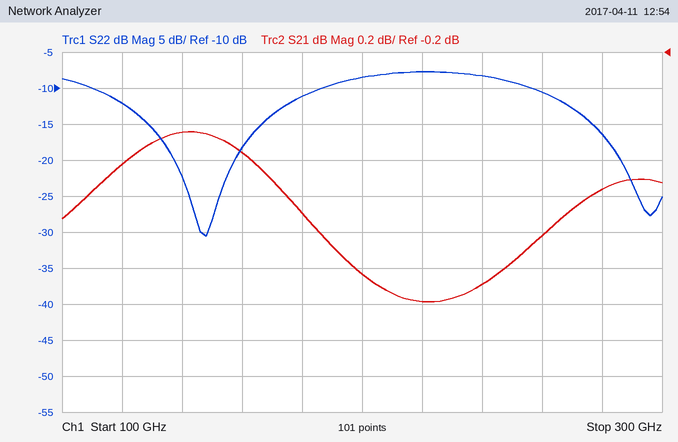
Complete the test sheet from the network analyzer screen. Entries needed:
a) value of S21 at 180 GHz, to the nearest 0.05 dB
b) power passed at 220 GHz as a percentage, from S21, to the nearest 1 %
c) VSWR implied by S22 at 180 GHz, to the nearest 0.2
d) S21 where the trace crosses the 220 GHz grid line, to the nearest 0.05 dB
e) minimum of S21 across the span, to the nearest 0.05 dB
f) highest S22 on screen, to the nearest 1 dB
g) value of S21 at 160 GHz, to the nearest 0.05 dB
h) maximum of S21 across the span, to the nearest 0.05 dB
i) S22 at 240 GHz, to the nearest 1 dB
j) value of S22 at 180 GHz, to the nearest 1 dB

-1.10 dB
69 %
1.8
-1.60 dB
-1.60 dB
-8 dB
-0.75 dB
-0.65 dB
-8 dB
-11 dB
